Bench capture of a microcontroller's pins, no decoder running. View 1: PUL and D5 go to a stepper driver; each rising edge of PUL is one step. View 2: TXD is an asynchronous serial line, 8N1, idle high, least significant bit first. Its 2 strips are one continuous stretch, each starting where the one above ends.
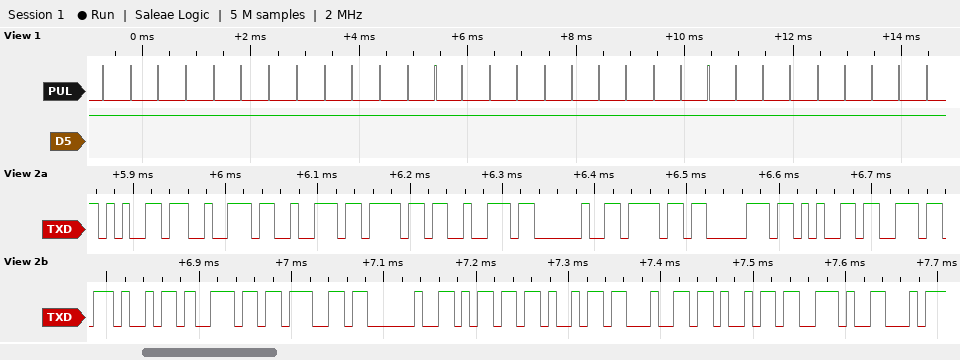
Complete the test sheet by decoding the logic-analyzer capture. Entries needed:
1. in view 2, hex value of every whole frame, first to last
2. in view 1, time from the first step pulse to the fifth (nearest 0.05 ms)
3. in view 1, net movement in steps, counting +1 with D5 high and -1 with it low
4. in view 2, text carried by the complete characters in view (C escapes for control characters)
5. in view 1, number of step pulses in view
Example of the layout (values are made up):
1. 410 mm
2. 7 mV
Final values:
1. 65 72 72 6F 72 20 6F 70 65 6E 69 6E 67 20 6D 69 64 69 2E
2. 2.05 ms
3. +31
4. "error opening midi."
5. 31
